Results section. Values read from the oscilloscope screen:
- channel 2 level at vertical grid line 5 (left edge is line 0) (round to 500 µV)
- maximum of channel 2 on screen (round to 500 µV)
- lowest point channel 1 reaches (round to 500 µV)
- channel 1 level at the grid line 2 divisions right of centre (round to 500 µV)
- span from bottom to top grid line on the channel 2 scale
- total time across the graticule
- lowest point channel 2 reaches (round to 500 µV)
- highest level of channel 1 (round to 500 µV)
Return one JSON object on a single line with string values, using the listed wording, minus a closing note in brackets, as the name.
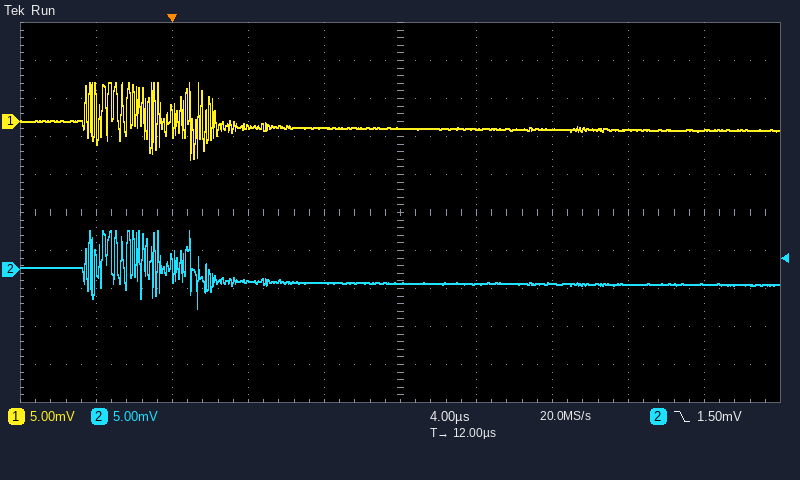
{"channel 2 level at vertical grid line 5 (left edge is line 0)": "-2.0 mV", "maximum of channel 2 on screen": "5.0 mV", "lowest point channel 1 reaches": "-5.0 mV", "channel 1 level at the grid line 2 divisions right of centre": "-1.0 mV", "span from bottom to top grid line on the channel 2 scale": "50 mV", "total time across the graticule": "40 µs", "lowest point channel 2 reaches": "-5.0 mV", "highest level of channel 1": "5.0 mV"}
